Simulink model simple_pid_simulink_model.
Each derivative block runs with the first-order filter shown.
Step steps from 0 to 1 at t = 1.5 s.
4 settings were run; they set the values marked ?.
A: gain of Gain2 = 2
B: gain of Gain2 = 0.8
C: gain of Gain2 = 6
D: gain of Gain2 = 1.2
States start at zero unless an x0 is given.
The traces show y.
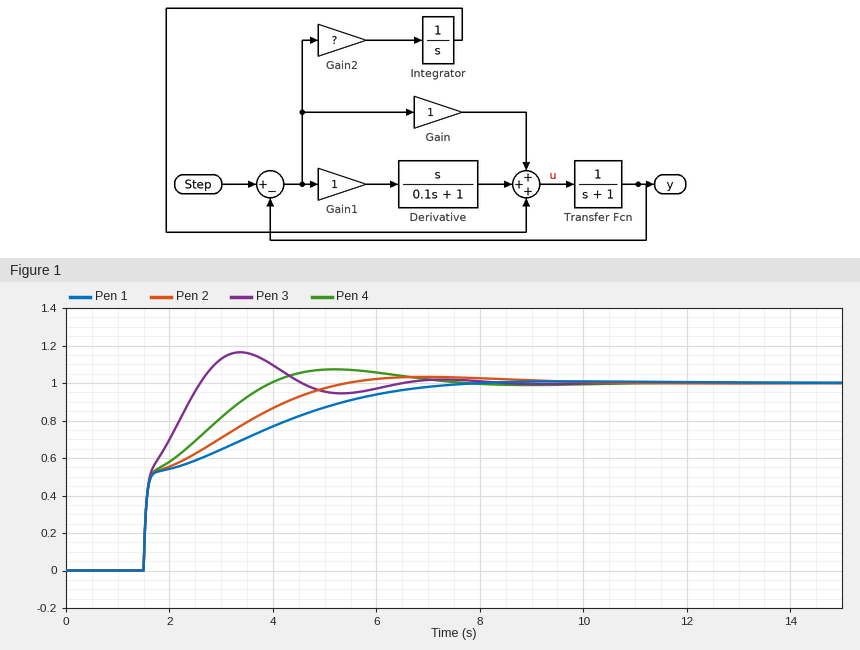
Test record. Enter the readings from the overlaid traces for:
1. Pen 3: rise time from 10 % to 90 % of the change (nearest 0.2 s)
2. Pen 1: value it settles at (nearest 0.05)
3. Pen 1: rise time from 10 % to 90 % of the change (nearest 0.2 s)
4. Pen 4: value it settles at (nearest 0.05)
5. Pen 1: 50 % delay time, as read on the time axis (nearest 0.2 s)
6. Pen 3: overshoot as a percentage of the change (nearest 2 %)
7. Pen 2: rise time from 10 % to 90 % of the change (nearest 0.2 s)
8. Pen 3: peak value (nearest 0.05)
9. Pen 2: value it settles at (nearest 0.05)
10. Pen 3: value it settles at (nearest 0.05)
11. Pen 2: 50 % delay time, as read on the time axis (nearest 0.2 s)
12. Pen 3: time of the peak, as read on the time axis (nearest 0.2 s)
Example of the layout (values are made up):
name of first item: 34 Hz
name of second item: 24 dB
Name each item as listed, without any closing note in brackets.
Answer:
Pen 3: rise time from 10 % to 90 % of the change: 0.8 s
Pen 1: value it settles at: 1.00
Pen 1: rise time from 10 % to 90 % of the change: 3.8 s
Pen 4: value it settles at: 1.00
Pen 1: 50 % delay time, as read on the time axis: 1.6 s
Pen 3: overshoot as a percentage of the change: 16 %
Pen 2: rise time from 10 % to 90 % of the change: 2.8 s
Pen 3: peak value: 1.15
Pen 2: value it settles at: 1.00
Pen 3: value it settles at: 1.00
Pen 2: 50 % delay time, as read on the time axis: 1.6 s
Pen 3: time of the peak, as read on the time axis: 3.4 s
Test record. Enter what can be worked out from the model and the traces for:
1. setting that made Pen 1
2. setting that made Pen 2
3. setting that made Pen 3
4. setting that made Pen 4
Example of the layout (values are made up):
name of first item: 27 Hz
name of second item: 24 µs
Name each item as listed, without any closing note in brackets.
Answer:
setting that made Pen 1: B
setting that made Pen 2: D
setting that made Pen 3: C
setting that made Pen 4: A
